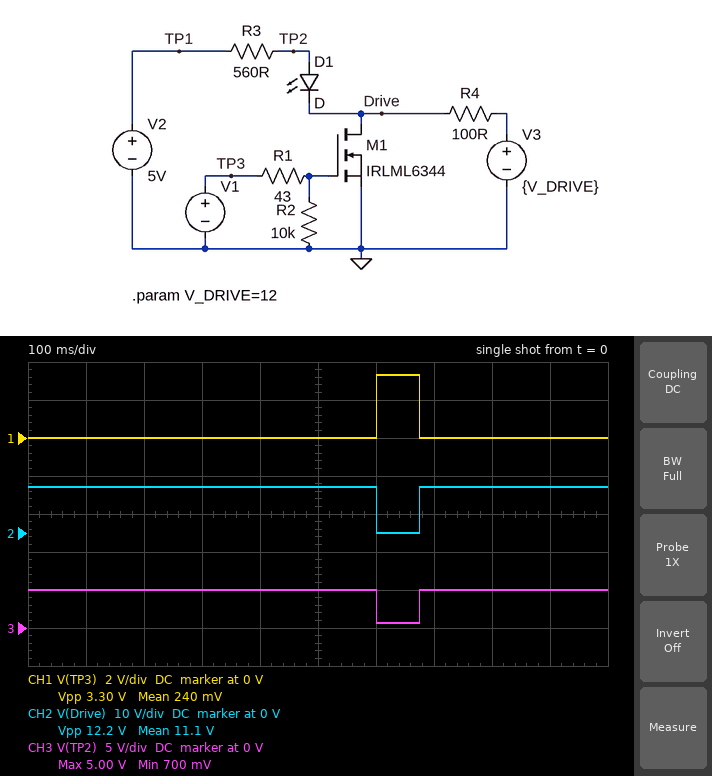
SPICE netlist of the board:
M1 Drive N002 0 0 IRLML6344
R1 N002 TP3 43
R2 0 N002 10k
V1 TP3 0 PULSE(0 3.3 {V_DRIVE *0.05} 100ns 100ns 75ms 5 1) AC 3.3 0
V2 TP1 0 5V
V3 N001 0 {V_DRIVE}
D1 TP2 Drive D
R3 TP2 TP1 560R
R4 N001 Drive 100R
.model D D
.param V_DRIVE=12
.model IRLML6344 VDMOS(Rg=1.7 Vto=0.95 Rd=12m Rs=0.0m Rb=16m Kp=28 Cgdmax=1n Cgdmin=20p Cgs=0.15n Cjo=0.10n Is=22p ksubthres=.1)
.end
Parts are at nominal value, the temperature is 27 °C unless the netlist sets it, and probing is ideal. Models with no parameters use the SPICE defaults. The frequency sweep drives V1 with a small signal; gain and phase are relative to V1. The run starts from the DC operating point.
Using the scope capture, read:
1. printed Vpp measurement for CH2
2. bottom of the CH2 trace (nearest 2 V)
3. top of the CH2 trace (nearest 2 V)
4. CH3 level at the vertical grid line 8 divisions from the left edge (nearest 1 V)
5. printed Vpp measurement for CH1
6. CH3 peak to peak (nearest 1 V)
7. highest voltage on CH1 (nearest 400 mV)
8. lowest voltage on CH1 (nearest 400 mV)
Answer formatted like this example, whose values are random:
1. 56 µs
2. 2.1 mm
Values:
1. 12.2 V
2. 0 V
3. 12 V
4. 5 V
5. 3.30 V
6. 4 V
7. 3.2 V
8. 0 V
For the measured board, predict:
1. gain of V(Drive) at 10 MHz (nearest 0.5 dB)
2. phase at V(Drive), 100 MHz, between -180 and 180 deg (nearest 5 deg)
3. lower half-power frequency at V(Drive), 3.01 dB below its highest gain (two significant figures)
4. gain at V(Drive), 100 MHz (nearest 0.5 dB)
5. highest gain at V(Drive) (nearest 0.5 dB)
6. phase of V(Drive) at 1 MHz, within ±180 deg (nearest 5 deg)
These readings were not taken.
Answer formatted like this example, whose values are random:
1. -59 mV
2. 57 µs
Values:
1. -12.0 dB
2. -65 deg
3. 8.1 MHz
4. -17.5 dB
5. -10.0 dB
6. 85 deg
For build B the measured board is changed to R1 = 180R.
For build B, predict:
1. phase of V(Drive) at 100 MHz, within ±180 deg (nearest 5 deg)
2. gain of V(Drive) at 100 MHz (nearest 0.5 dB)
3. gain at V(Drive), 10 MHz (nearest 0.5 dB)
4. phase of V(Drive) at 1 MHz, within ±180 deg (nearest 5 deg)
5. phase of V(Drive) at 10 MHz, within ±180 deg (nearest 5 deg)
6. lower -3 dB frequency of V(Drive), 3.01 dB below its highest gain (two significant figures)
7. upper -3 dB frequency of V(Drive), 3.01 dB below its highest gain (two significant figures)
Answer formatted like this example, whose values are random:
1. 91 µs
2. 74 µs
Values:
1. -75 deg
2. -29.5 dB
3. -18.5 dB
4. 75 deg
5. 0 deg
6. 3.3 MHz
7. 34 MHz
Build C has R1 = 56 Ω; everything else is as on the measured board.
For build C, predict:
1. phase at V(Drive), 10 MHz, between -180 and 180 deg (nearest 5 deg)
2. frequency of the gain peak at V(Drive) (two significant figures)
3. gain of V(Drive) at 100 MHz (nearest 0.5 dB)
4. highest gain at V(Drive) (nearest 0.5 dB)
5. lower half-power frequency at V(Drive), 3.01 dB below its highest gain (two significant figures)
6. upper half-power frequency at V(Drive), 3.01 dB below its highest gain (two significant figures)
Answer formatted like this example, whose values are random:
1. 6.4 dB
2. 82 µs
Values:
1. 30 deg
2. 19 MHz
3. -19.5 dB
4. -11.5 dB
5. 7.1 MHz
6. 49 MHz
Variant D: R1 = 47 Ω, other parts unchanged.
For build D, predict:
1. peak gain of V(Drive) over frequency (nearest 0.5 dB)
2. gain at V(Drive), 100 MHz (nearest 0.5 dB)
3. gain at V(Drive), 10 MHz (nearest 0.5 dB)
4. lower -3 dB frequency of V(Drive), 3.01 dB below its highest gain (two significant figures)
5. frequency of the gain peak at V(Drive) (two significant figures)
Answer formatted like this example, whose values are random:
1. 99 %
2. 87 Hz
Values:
1. -10.5 dB
2. -18.0 dB
3. -12.5 dB
4. 7.8 MHz
5. 20 MHz
